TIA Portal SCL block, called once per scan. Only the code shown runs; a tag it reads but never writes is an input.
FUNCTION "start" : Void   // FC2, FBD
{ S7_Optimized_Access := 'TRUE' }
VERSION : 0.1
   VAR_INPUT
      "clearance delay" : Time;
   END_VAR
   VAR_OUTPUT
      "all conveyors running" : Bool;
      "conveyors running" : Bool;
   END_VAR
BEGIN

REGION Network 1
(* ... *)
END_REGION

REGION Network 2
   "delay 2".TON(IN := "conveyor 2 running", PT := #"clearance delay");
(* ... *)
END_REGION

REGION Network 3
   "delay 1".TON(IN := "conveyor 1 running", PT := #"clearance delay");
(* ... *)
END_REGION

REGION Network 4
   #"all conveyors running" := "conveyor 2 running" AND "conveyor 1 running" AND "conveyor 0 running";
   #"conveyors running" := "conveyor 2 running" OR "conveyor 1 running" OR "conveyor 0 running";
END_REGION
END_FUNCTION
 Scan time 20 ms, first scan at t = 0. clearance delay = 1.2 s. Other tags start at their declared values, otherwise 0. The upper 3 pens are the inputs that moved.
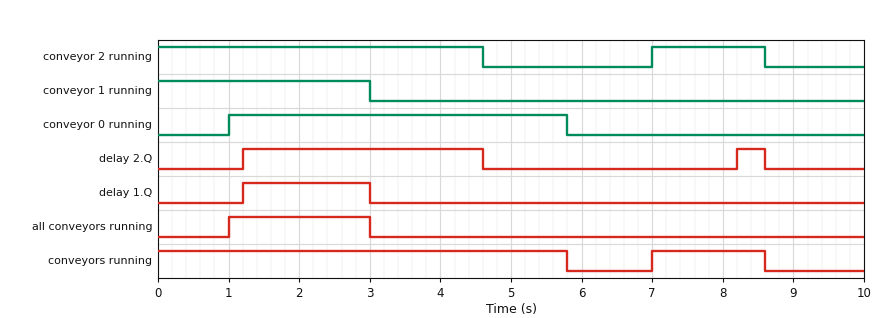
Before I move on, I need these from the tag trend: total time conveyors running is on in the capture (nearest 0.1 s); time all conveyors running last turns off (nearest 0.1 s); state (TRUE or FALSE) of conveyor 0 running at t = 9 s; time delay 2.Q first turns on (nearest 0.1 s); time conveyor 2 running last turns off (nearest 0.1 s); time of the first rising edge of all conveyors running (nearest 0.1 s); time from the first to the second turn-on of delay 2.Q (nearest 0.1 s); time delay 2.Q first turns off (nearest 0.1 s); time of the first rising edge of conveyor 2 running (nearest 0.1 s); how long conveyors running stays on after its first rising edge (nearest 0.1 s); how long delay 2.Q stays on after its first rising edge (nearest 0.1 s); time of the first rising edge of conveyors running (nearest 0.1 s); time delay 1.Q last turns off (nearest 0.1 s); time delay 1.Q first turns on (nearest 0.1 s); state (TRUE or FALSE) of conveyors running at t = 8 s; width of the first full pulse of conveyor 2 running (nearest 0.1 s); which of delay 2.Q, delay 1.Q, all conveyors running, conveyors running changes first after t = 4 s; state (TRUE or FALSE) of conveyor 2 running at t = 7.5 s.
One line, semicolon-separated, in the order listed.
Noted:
7.4 s; 3.0 s; FALSE; 1.2 s; 8.6 s; 1.0 s; 7.0 s; 4.6 s; 7.0 s; 1.6 s; 3.4 s; 7.0 s; 3.0 s; 1.2 s; TRUE; 1.6 s; delay 2.Q; TRUE
